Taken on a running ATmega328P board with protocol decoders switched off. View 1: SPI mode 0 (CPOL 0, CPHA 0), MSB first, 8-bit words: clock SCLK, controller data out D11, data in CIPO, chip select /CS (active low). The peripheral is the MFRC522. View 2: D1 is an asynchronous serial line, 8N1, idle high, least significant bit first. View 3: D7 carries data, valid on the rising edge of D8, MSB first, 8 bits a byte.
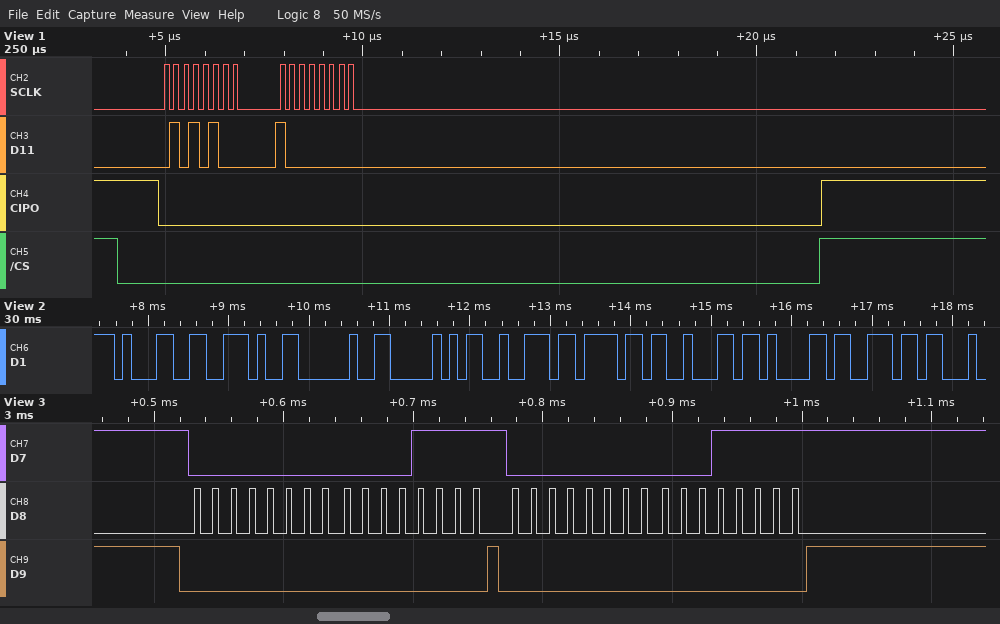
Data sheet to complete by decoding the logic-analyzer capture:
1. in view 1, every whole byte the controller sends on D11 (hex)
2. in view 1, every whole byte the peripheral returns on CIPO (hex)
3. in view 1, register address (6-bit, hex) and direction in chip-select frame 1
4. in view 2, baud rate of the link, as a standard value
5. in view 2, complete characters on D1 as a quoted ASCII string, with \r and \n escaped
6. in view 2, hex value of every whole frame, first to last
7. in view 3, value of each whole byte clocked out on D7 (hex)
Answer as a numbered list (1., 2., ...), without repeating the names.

1. 54 80
2. 00 00
3. 0x2A write
4. 9600 baud
5. "1. Proban"
6. 31 2E 20 50 72 6F 62 61 6E
7. 00 0F 00 1F
